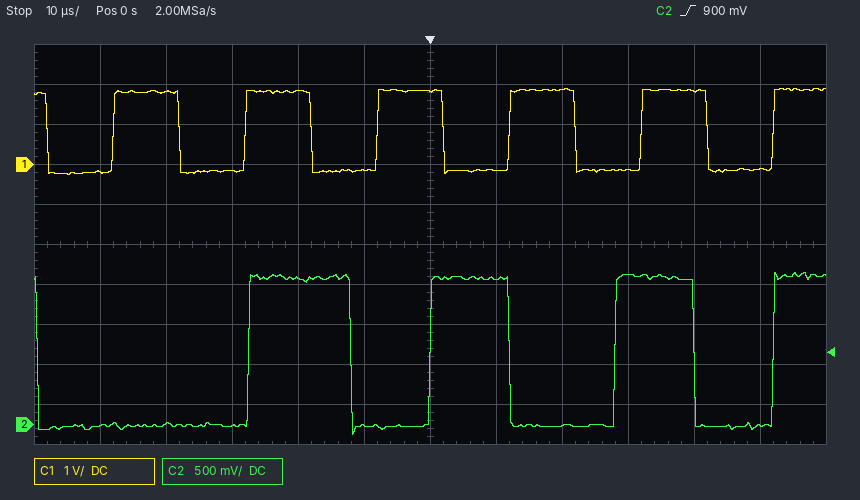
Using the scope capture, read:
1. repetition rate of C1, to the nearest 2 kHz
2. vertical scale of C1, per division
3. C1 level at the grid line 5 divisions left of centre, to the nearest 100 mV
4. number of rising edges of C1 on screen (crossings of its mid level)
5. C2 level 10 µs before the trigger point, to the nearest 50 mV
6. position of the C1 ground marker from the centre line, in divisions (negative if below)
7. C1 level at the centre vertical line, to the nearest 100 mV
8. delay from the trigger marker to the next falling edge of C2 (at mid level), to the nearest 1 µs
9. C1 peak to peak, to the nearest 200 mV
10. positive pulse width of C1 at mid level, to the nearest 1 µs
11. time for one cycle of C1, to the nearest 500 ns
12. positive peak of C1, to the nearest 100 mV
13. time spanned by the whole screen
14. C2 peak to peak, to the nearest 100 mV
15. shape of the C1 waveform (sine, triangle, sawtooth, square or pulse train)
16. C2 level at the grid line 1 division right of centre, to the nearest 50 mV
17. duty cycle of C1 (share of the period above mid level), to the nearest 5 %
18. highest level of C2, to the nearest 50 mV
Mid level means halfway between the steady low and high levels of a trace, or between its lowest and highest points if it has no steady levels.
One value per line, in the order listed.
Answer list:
50 kHz
1 V
-200 mV
6
0 mV
+2.0 div
1.8 V
12 µs
2.2 V
10 µs
20.0 µs
1.9 V
120 µs
2.00 V
square
1.80 V
50 %
1.90 V
